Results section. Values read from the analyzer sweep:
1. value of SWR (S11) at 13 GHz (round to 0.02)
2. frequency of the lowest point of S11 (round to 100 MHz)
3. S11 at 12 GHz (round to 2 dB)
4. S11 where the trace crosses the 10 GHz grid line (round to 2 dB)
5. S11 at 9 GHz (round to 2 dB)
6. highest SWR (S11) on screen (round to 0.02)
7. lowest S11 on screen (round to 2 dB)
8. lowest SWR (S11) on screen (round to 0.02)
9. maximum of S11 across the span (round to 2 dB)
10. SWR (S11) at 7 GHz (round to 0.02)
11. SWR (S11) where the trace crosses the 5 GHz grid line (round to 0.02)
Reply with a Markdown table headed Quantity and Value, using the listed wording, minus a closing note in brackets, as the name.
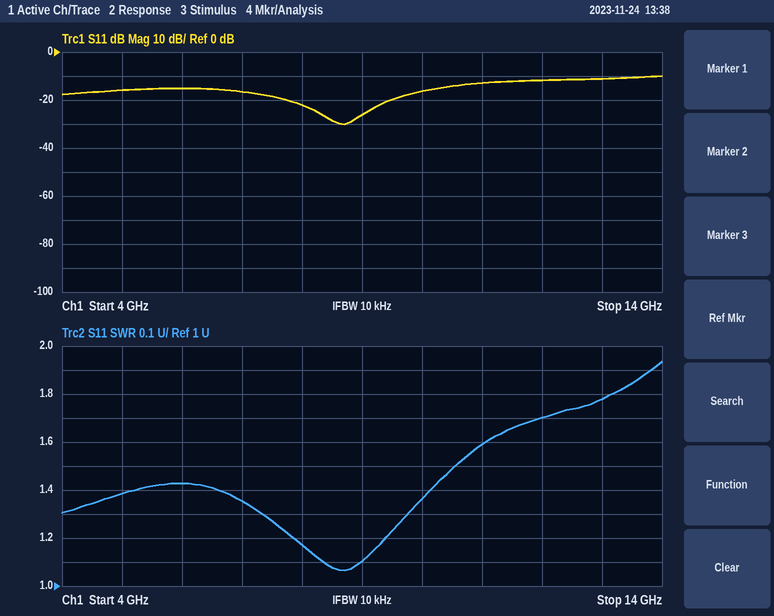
| Quantity | Value |
|---|---|
| value of SWR (S11) at 13 GHz | 1.78 |
| frequency of the lowest point of S11 | 8.7 GHz |
| S11 at 12 GHz | -12 dB |
| S11 where the trace crosses the 10 GHz grid line | -16 dB |
| S11 at 9 GHz | -26 dB |
| highest SWR (S11) on screen | 1.94 |
| lowest S11 on screen | -30 dB |
| lowest SWR (S11) on screen | 1.06 |
| maximum of S11 across the span | -10 dB |
| SWR (S11) at 7 GHz | 1.36 |
| SWR (S11) where the trace crosses the 5 GHz grid line | 1.38 |
